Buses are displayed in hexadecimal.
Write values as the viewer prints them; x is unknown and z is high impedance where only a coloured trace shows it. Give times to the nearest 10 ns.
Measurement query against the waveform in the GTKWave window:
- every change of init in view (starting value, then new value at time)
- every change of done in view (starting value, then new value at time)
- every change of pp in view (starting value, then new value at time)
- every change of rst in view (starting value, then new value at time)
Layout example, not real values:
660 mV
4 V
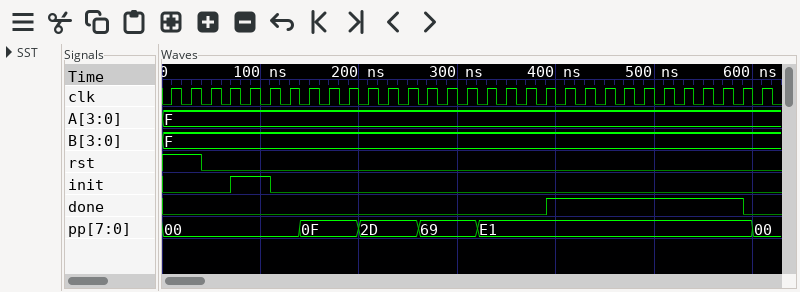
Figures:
0, 1 at 70 ns, 0 at 110 ns
0, 1 at 390 ns, 0 at 590 ns
00, 0F at 140 ns, 2D at 200 ns, 69 at 260 ns, E1 at 320 ns, 00 at 600 ns
1, 0 at 40 ns
